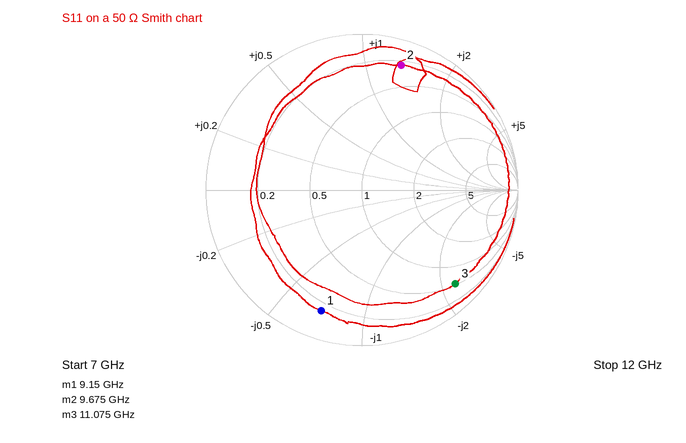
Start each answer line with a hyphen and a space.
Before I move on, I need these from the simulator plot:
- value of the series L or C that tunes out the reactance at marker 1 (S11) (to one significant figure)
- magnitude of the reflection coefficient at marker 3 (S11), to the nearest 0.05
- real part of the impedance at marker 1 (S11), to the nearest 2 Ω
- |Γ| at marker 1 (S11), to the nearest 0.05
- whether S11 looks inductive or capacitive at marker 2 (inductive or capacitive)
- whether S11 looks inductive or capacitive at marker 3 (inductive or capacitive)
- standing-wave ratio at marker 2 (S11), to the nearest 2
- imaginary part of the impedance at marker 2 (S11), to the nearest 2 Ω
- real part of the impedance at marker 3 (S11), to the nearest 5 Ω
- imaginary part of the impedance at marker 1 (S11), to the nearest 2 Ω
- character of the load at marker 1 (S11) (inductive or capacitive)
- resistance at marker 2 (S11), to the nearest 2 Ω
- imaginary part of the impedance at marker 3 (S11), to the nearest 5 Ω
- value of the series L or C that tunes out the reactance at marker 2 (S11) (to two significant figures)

- 600 pH
- 0.85
- 8 Ω
- 0.80
- inductive
- capacitive
- 12
- +66 Ω
- 25 Ω
- -36 Ω
- capacitive
- 12 Ω
- -115 Ω
- 250 fF
